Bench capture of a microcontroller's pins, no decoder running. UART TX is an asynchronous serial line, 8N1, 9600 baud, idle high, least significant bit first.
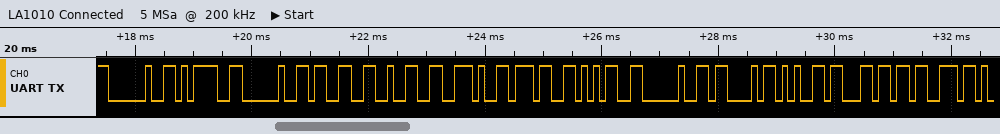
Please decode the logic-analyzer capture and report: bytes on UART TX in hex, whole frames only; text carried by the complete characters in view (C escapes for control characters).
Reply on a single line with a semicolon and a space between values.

0x20 0x3D 0x20 0x33 0x32 0x2E 0x37 0x35 0x20 0x43 0x65 0x6C 0x73; " = 32.75 Cels"
